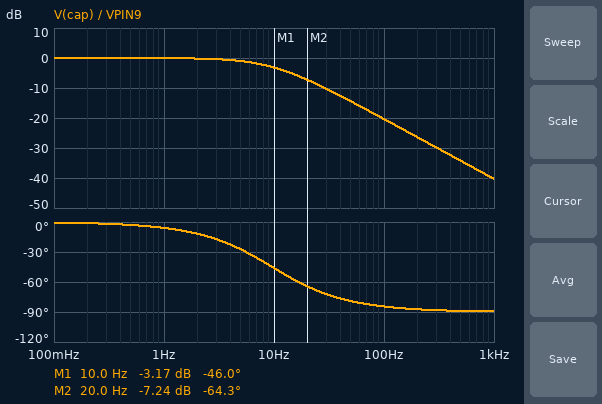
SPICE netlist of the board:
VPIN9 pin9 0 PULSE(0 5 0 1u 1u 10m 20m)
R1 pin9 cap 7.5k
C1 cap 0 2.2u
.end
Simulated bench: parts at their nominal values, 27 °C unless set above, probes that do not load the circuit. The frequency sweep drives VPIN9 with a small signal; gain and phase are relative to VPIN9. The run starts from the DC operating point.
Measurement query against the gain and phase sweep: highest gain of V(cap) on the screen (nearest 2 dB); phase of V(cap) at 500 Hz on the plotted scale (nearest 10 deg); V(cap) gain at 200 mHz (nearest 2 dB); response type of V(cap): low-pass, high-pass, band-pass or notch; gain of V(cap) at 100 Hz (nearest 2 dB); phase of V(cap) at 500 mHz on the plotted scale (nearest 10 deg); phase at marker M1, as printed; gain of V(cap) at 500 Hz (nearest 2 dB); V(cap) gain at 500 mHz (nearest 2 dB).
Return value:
0 dB
-90 deg
0 dB
low-pass
-20 dB
0 deg
-46.0 deg
-34 dB
0 dB
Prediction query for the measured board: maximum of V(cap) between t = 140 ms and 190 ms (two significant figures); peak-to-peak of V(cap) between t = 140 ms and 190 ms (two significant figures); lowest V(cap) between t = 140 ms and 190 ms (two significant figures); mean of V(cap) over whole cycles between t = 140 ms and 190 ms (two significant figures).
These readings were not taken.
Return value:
3.2 V
1.5 V
1.8 V
2.5 V
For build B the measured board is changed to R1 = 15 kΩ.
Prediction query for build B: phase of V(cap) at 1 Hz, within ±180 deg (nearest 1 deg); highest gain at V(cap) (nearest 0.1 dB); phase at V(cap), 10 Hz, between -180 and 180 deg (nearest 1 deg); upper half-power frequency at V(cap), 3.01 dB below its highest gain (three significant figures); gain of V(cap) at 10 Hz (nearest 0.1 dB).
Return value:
-12 deg
0 dB
-64 deg
4.82 Hz
-7.2 dB
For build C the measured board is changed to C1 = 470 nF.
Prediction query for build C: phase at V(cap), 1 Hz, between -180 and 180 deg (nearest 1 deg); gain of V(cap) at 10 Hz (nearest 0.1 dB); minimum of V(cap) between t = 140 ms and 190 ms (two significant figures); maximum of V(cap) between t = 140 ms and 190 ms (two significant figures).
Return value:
-1 deg
-0.2 dB
280 mV
4.7 V
